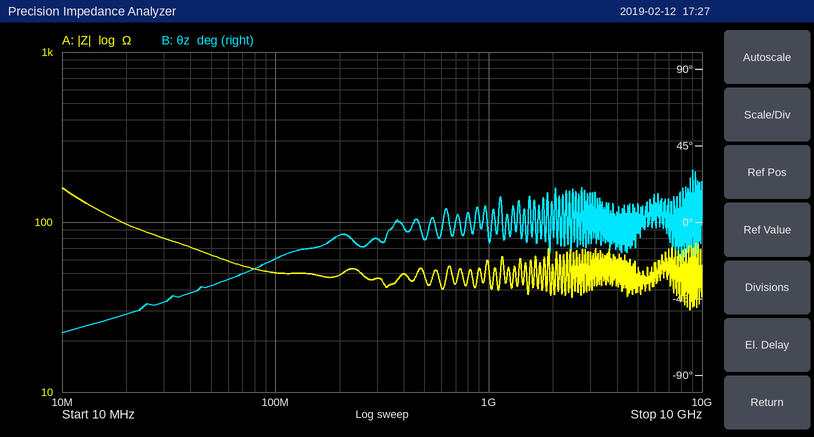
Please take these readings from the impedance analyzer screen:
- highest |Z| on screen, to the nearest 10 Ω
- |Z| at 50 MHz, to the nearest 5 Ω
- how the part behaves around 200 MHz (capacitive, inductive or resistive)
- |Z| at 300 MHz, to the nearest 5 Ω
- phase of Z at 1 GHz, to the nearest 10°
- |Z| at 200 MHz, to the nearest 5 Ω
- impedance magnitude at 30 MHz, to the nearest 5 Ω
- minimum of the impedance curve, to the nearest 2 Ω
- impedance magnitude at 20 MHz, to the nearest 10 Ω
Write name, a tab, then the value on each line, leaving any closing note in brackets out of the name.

highest |Z| on screen, to the nearest 10 Ω	160 Ω
|Z| at 50 MHz, to the nearest 5 Ω	65 Ω
how the part behaves around 200 MHz	resistive
|Z| at 300 MHz, to the nearest 5 Ω	45 Ω
phase of Z at 1 GHz, to the nearest 10°	-10°
|Z| at 200 MHz, to the nearest 5 Ω	50 Ω
impedance magnitude at 30 MHz, to the nearest 5 Ω	80 Ω
minimum of the impedance curve, to the nearest 2 Ω	30 Ω
impedance magnitude at 20 MHz, to the nearest 10 Ω	100 Ω
